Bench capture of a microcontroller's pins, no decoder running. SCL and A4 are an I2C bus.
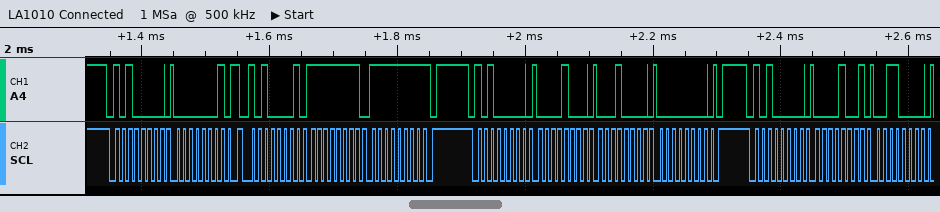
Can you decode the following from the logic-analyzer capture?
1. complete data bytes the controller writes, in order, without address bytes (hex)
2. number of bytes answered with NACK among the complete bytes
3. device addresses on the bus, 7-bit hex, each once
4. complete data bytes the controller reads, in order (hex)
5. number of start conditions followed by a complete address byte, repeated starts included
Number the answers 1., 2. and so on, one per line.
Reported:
1. 01 08 10 00 09 30
2. 1
3. 0x50
4. FF FF
5. 4
